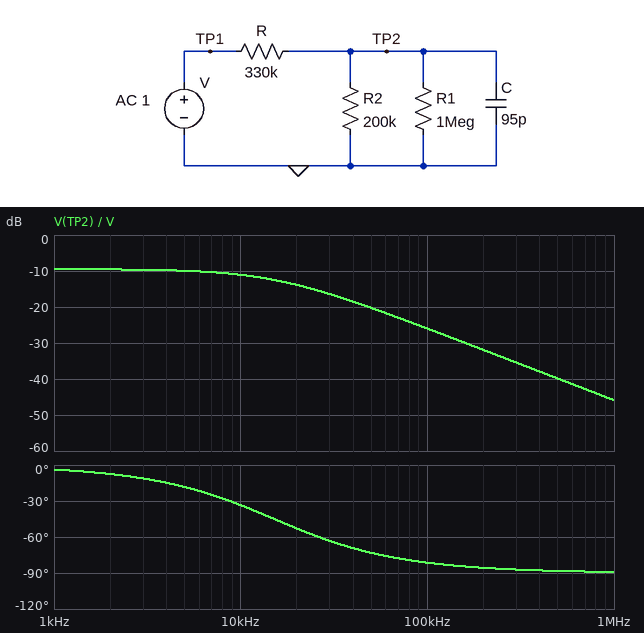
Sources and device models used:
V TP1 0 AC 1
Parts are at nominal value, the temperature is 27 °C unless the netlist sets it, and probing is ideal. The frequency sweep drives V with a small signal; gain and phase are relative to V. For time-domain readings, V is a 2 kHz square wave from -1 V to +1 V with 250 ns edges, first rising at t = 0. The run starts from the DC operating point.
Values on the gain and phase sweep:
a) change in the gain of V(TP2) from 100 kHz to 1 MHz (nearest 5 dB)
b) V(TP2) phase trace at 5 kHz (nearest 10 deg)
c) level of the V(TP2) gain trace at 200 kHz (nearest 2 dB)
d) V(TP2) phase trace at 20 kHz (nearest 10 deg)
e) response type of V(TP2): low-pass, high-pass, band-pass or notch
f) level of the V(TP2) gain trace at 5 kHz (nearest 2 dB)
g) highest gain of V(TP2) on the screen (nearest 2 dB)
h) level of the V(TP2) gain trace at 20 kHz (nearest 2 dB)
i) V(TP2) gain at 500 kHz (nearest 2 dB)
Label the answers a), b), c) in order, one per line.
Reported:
a) -20 dB
b) -20 deg
c) -32 dB
d) -50 deg
e) low-pass
f) -10 dB
g) -10 dB
h) -14 dB
i) -40 dB
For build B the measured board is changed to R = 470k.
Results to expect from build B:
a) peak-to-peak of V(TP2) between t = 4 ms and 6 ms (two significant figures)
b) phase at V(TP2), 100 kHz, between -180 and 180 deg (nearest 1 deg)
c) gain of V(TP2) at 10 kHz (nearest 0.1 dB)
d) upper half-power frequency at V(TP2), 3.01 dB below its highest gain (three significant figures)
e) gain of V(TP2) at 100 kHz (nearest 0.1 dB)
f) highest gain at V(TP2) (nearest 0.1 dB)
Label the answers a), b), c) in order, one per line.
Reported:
a) 520 mV
b) -82 deg
c) -13.5 dB
d) 13.6 kHz
e) -29.0 dB
f) -11.6 dB
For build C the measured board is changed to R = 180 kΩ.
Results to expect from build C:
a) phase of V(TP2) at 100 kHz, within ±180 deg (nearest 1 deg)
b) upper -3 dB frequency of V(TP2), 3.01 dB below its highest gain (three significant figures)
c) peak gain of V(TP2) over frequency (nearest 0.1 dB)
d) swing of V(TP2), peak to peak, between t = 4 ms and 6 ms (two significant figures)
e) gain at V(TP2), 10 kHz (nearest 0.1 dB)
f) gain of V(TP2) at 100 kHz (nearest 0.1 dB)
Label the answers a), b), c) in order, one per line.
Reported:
a) -79 deg
b) 19.4 kHz
c) -6.4 dB
d) 960 mV
e) -7.4 dB
f) -20.8 dB
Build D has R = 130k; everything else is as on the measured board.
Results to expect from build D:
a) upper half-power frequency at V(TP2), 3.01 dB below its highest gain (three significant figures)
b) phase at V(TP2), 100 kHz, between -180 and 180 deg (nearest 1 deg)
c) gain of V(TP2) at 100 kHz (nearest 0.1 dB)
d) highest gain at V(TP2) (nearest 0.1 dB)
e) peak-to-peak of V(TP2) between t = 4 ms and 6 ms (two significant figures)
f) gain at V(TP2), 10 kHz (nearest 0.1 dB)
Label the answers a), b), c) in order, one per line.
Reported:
a) 22.9 kHz
b) -77 deg
c) -18.0 dB
d) -5.0 dB
e) 1.1 V
f) -5.8 dB
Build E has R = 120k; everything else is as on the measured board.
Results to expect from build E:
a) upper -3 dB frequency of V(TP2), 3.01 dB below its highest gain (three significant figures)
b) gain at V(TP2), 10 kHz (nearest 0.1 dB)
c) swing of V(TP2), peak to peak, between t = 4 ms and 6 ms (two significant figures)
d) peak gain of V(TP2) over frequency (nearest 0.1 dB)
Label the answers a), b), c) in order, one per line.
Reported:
a) 24.0 kHz
b) -5.4 dB
c) 1.2 V
d) -4.7 dB
